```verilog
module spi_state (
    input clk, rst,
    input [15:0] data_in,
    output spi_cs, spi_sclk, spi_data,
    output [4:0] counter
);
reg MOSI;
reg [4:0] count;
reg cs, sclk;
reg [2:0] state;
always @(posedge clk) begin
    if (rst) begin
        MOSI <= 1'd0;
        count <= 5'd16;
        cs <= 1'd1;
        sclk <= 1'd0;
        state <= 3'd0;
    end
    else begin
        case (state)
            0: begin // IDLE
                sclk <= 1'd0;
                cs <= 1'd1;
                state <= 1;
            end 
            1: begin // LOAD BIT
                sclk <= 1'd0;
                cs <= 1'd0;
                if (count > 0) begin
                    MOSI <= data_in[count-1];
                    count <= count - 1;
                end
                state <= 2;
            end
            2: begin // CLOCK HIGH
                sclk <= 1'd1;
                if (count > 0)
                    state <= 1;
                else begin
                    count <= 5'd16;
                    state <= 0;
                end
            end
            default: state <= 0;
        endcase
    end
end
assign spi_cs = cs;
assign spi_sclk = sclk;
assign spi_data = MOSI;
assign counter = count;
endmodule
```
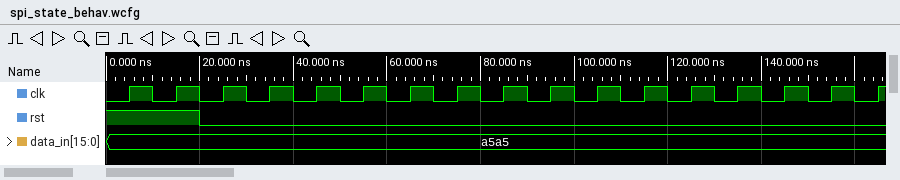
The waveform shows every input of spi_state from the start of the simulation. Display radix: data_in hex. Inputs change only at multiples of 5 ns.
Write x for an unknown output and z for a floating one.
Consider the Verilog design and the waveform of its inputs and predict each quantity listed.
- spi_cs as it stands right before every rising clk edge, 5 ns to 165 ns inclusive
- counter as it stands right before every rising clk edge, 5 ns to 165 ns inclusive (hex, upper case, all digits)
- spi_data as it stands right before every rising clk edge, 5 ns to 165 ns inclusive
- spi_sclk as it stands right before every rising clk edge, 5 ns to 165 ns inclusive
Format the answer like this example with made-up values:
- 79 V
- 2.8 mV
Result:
- x 1 1 1 0 0 0 0 0 0 0 0 0 0 0 0 0
- x, 10, 10, 10, 0F, 0F, 0E, 0E, 0D, 0D, 0C, 0C, 0B, 0B, 0A, 0A, 09
- x 0 0 0 1 1 0 0 1 1 0 0 0 0 1 1 0
- x 0 0 0 0 1 0 1 0 1 0 1 0 1 0 1 0
